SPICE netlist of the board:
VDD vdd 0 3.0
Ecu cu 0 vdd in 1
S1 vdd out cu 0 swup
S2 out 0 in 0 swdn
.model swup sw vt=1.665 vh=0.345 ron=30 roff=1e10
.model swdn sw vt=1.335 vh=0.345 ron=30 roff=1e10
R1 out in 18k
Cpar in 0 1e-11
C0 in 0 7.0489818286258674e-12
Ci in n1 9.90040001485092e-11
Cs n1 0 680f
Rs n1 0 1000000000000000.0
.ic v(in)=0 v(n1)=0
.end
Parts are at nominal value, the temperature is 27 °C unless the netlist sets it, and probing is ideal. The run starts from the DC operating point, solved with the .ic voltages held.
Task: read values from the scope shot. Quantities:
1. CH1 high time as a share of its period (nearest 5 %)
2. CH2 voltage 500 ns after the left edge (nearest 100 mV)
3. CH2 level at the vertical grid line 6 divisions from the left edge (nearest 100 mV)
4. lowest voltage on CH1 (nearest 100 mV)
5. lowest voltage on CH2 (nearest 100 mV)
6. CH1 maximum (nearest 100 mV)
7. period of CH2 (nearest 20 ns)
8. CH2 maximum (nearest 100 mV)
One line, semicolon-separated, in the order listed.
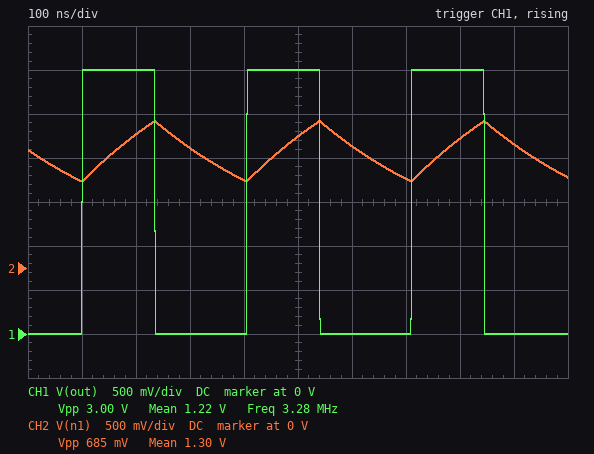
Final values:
45 %; 1.5 V; 1.4 V; 0 V; 1.0 V; 3.0 V; 300 ns; 1.7 V
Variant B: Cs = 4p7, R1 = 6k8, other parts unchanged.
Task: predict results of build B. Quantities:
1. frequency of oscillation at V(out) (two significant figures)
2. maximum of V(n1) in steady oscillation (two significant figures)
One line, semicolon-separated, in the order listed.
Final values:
7.2 MHz; 1.6 V
